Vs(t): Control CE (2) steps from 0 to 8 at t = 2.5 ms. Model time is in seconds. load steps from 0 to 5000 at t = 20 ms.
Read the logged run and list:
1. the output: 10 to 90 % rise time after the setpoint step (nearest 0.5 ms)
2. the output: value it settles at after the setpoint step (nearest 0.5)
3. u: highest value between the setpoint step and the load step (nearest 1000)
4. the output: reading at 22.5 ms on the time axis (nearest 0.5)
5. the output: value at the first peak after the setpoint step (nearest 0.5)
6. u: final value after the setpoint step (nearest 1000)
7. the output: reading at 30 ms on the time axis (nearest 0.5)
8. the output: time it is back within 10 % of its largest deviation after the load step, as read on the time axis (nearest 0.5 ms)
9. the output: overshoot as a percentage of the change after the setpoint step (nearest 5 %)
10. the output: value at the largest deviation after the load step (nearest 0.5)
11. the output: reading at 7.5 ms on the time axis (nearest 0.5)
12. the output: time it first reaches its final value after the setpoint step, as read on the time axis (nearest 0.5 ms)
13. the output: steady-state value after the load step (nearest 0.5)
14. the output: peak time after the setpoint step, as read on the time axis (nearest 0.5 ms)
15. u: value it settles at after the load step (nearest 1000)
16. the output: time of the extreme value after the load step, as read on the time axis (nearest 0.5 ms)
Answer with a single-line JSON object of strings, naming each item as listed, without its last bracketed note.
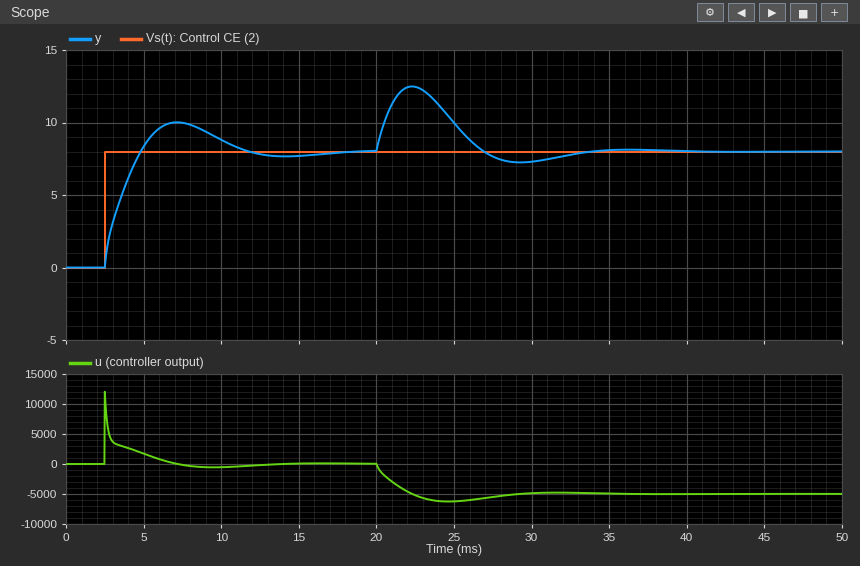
{"the output: 10 to 90 % rise time after the setpoint step": "2.0 ms", "the output: value it settles at after the setpoint step": "8.0", "u: highest value between the setpoint step and the load step": "12000", "the output: reading at 22.5 ms on the time axis": "12.5", "the output: value at the first peak after the setpoint step": "10.0", "u: final value after the setpoint step": "0", "the output: reading at 30 ms on the time axis": "7.5", "the output: time it is back within 10 % of its largest deviation after the load step, as read on the time axis": "31.5 ms", "the output: overshoot as a percentage of the change after the setpoint step": "25 %", "the output: value at the largest deviation after the load step": "12.5", "the output: reading at 7.5 ms on the time axis": "10.0", "the output: time it first reaches its final value after the setpoint step, as read on the time axis": "5.0 ms", "the output: steady-state value after the load step": "8.0", "the output: peak time after the setpoint step, as read on the time axis": "7.0 ms", "u: value it settles at after the load step": "-5000", "the output: time of the extreme value after the load step, as read on the time axis": "22.5 ms"}
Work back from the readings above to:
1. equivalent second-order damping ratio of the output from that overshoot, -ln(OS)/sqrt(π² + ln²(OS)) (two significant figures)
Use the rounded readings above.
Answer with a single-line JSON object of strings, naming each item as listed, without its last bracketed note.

{"equivalent second-order damping ratio of the output from that overshoot, -ln(OS)/sqrt(π² + ln²(OS))": "0.40"}
